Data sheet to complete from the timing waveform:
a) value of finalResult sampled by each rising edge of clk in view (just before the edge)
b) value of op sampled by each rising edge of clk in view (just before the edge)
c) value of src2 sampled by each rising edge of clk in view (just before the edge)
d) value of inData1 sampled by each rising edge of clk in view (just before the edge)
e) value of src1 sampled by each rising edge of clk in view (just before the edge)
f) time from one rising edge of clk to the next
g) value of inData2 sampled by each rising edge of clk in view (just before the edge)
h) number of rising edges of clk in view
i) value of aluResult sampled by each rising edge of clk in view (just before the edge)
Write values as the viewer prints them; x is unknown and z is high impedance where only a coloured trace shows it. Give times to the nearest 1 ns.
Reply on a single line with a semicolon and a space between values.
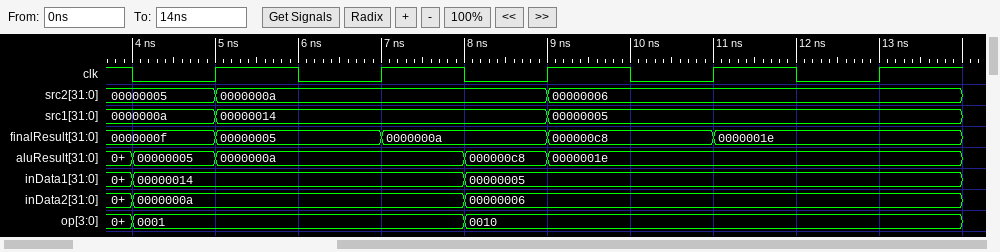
0000000f, 00000005, 0000000a, 000000c8, 0000001e; 0001, 0001, 0010, 0010, 0010; 00000005, 0000000a, 0000000a, 00000006, 00000006; 00000014, 00000014, 00000005, 00000005, 00000005; 0000000a, 00000014, 00000014, 00000005, 00000005; 2 ns; 0000000a, 0000000a, 00000006, 00000006, 00000006; 5; 00000005, 0000000a, 000000c8, 0000001e, 0000001e
